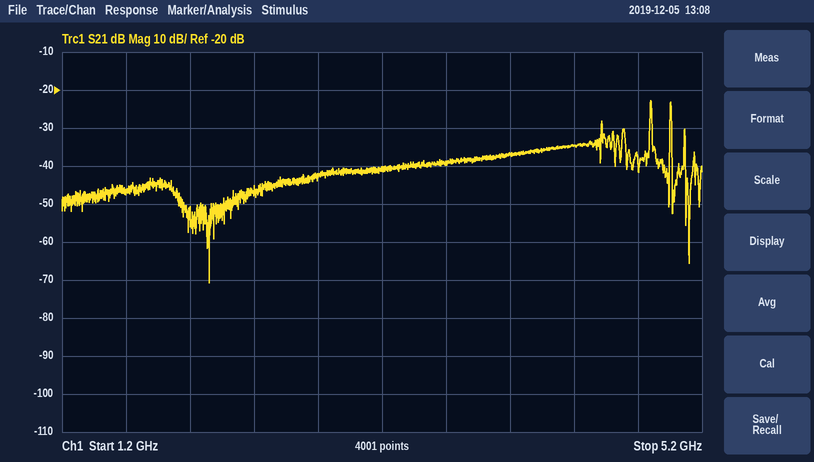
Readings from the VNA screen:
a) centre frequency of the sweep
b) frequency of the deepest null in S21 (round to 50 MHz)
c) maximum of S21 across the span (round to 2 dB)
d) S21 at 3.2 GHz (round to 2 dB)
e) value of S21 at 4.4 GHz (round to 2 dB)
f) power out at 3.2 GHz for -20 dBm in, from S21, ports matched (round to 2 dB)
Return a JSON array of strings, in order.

["3.2 GHz", "2.10 GHz", "-22 dB", "-40 dB", "-34 dB", "-60 dBm"]
